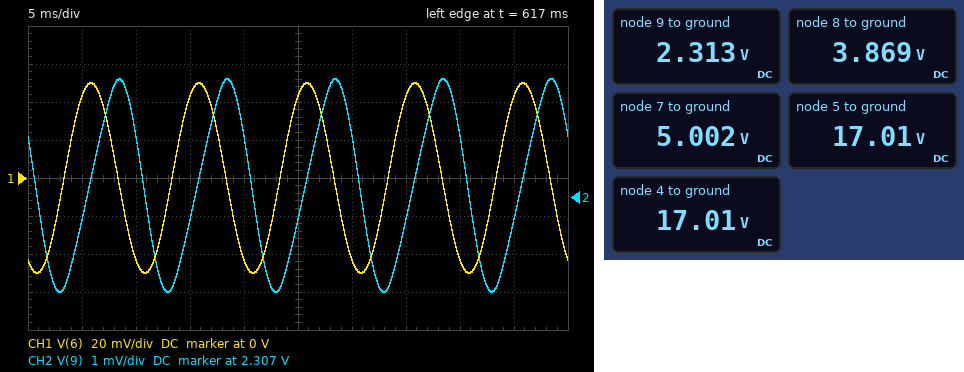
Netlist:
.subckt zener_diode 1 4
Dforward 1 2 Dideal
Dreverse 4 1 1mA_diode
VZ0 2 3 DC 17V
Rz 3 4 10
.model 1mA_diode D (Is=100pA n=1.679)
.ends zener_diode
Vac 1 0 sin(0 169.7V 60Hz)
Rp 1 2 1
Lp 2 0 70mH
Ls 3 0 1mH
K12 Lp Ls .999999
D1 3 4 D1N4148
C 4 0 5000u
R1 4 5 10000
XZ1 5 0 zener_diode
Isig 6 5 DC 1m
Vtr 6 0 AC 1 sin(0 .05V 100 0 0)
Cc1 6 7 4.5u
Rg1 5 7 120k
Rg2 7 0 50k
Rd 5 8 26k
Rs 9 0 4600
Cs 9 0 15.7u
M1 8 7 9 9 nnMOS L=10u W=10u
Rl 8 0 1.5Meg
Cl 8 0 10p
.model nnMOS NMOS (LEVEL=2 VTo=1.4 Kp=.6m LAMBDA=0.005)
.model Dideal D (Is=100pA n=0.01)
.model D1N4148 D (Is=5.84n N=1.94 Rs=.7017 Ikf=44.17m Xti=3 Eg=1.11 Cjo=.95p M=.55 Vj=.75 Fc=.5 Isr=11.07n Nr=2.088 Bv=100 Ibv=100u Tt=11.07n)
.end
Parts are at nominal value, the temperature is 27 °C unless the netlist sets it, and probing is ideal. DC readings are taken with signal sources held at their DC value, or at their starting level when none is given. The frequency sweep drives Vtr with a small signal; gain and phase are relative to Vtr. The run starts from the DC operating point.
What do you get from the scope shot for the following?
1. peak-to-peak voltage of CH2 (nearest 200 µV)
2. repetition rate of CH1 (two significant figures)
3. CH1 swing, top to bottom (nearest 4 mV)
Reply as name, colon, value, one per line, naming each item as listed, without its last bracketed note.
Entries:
peak-to-peak voltage of CH2: 5.6 mV
repetition rate of CH1: 100 Hz
CH1 swing, top to bottom: 100 mV
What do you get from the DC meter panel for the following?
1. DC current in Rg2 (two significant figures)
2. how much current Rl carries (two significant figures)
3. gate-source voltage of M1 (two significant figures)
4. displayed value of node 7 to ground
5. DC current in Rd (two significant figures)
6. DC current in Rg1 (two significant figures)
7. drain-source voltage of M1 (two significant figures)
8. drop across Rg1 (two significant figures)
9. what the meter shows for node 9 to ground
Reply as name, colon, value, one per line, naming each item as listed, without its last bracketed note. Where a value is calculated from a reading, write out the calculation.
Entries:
DC current in Rg2: (5.002 V) / 50 kΩ = 100 µA
how much current Rl carries: (3.869 V) / 1.5 MΩ = 2.6 µA
gate-source voltage of M1: 5.002 V - 2.313 V = 2.7 V
displayed value of node 7 to ground: 5.002 V
DC current in Rd: (17.01 V - 3.869 V) / 26 kΩ = 510 µA
DC current in Rg1: (17.01 V - 5.002 V) / 120 kΩ = 100 µA
drain-source voltage of M1: 3.869 V - 2.313 V = 1.6 V
drop across Rg1: 17.01 V - 5.002 V = 12 V
what the meter shows for node 9 to ground: 2.313 V
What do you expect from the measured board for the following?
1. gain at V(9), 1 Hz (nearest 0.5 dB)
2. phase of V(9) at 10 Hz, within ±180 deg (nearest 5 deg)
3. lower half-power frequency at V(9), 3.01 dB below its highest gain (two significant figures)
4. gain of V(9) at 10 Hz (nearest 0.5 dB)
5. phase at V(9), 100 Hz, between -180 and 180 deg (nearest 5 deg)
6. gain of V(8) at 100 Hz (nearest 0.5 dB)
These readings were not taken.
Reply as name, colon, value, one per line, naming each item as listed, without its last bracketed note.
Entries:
gain at V(9), 1 Hz: -5.5 dB
phase of V(9) at 10 Hz, within ±180 deg: -40 deg
lower half-power frequency at V(9), 3.01 dB below its highest gain: 840 mHz
gain of V(9) at 10 Hz: -5.5 dB
phase at V(9), 100 Hz, between -180 and 180 deg: -85 deg
gain of V(8) at 100 Hz: 25.5 dB
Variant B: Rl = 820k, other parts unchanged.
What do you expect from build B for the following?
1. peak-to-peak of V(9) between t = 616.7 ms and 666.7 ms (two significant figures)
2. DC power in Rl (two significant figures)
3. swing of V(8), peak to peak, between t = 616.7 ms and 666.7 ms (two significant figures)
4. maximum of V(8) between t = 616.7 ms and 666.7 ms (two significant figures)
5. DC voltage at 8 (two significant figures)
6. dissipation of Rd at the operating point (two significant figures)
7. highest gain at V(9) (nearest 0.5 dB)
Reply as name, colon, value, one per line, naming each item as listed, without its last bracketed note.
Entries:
peak-to-peak of V(9) between t = 616.7 ms and 666.7 ms: 5.4 mV
DC power in Rl: 18 µW
swing of V(8), peak to peak, between t = 616.7 ms and 666.7 ms: 1.2 V
maximum of V(8) between t = 616.7 ms and 666.7 ms: 4.6 V
DC voltage at 8: 3.8 V
dissipation of Rd at the operating point: 6.7 mW
highest gain at V(9): -3.0 dB
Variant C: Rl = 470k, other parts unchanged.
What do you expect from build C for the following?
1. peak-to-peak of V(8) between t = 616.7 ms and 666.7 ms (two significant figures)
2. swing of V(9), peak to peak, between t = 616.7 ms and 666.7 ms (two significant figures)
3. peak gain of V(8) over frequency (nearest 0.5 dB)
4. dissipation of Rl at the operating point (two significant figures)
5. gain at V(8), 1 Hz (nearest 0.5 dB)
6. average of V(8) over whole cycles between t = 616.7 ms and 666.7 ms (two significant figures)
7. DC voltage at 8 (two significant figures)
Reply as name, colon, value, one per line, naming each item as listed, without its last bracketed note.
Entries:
peak-to-peak of V(8) between t = 616.7 ms and 666.7 ms: 1.1 V
swing of V(9), peak to peak, between t = 616.7 ms and 666.7 ms: 5.0 mV
peak gain of V(8) over frequency: 25.0 dB
dissipation of Rl at the operating point: 30 µW
gain at V(8), 1 Hz: 10.0 dB
average of V(8) over whole cycles between t = 616.7 ms and 666.7 ms: 3.8 V
DC voltage at 8: 3.7 V
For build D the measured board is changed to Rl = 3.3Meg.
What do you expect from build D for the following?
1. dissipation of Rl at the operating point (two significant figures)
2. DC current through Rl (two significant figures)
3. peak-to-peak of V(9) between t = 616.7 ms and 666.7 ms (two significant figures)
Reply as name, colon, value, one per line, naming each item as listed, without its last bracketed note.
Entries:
dissipation of Rl at the operating point: 4.6 µW
DC current through Rl: 1.2 µA
peak-to-peak of V(9) between t = 616.7 ms and 666.7 ms: 5.8 mV
